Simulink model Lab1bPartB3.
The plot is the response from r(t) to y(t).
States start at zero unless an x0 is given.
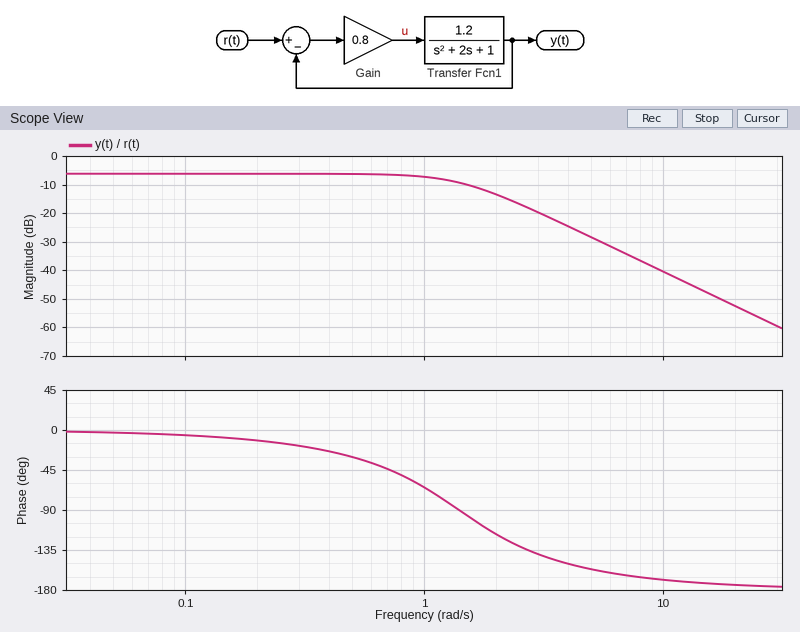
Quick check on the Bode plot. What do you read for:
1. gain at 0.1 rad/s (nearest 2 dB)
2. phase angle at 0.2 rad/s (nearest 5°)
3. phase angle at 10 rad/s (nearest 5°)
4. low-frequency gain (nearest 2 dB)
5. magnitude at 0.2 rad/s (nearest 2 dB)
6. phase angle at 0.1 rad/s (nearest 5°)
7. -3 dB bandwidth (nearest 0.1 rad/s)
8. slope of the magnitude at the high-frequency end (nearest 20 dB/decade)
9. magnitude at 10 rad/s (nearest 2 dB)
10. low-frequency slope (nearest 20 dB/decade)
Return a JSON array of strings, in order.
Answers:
["-6 dB", "-10°", "-170°", "-6 dB", "-6 dB", "-5°", "1.4 rad/s", "-40 dB/decade", "-40 dB", "0 dB/decade"]
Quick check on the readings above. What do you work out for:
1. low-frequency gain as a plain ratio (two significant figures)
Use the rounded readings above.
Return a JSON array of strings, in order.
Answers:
["0.50"]
